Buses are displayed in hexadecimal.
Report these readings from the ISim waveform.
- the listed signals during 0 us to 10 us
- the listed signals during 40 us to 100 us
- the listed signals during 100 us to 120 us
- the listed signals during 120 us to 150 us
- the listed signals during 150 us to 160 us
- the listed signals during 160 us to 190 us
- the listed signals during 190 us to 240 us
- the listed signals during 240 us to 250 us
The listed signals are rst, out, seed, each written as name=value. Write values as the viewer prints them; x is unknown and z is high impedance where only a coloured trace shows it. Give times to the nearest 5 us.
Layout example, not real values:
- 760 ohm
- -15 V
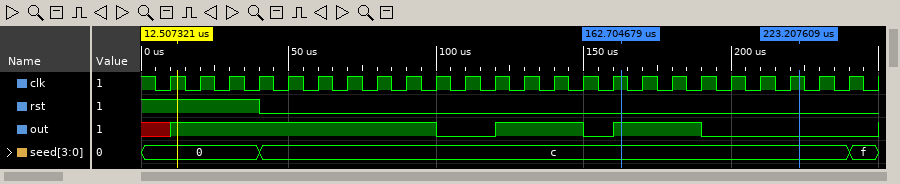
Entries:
- rst=1, out=x, seed=0
- rst=0, out=1, seed=c
- rst=0, out=0, seed=c
- rst=0, out=1, seed=c
- rst=0, out=0, seed=c
- rst=0, out=1, seed=c
- rst=0, out=0, seed=c
- rst=0, out=0, seed=f
